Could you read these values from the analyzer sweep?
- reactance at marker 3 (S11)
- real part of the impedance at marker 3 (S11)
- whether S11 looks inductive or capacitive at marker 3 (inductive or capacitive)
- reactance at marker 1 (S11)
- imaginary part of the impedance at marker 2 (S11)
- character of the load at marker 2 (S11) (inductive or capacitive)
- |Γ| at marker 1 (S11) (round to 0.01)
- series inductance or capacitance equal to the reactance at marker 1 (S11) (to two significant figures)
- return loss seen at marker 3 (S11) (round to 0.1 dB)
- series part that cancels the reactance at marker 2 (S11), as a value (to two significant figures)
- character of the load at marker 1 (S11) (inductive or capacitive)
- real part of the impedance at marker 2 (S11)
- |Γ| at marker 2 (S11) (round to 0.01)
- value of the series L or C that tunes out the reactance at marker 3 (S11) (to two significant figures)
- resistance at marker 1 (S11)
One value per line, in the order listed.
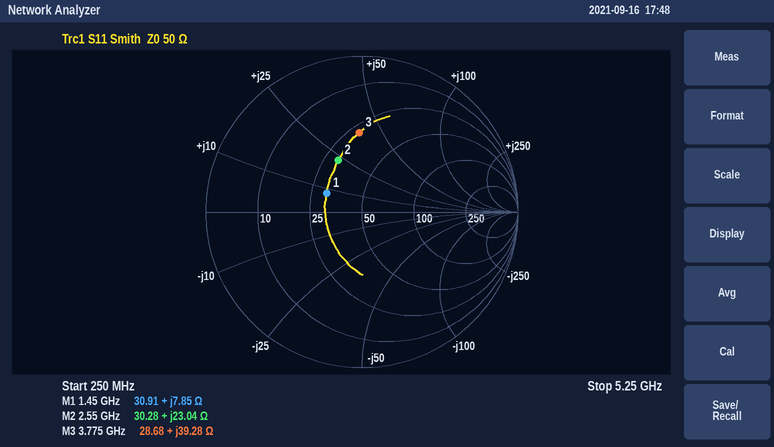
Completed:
+39.28 Ω
28.68 Ω
inductive
+7.85 Ω
+23.04 Ω
inductive
0.25
860 pH
5.9 dB
2.7 pF
inductive
30.28 Ω
0.36
1.1 pF
30.91 Ω
